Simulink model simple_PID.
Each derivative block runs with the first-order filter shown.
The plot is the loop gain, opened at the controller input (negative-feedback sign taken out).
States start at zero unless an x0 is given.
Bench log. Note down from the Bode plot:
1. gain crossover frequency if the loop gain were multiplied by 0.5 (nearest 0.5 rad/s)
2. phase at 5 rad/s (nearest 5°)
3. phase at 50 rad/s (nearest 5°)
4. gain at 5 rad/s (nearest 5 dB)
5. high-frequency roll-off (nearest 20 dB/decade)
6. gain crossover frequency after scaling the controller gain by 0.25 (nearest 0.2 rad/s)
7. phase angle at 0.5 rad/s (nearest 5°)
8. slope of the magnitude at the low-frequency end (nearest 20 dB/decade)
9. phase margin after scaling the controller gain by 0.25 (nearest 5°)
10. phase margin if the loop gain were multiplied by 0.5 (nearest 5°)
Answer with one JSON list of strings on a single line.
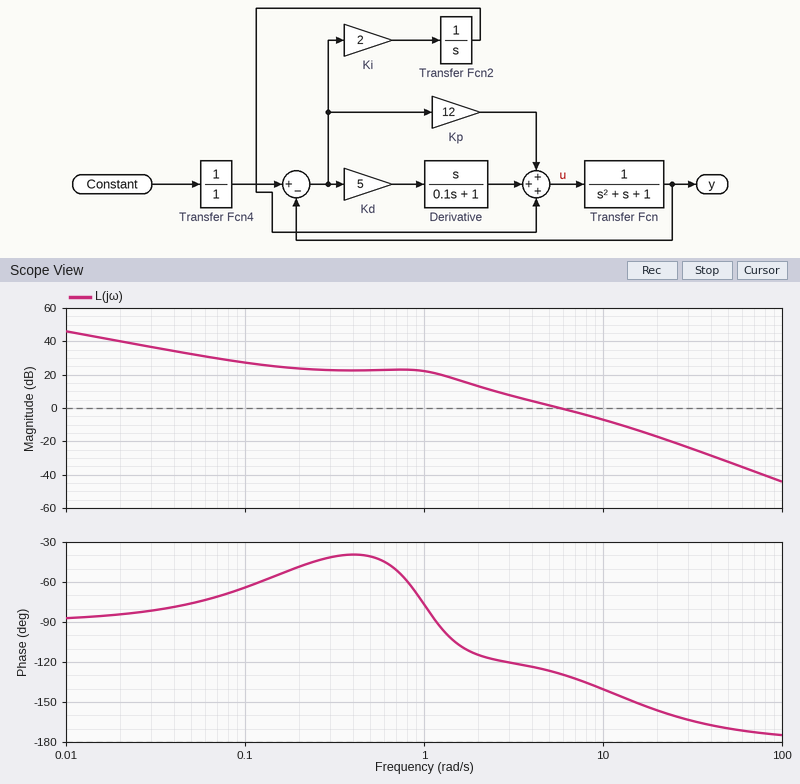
["3.5 rad/s", "-125°", "-170°", "0 dB", "-40 dB/decade", "2.2 rad/s", "-40°", "-20 dB/decade", "65°", "60°"]
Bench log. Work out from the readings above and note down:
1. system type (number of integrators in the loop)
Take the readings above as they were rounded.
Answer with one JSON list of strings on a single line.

["1"]
